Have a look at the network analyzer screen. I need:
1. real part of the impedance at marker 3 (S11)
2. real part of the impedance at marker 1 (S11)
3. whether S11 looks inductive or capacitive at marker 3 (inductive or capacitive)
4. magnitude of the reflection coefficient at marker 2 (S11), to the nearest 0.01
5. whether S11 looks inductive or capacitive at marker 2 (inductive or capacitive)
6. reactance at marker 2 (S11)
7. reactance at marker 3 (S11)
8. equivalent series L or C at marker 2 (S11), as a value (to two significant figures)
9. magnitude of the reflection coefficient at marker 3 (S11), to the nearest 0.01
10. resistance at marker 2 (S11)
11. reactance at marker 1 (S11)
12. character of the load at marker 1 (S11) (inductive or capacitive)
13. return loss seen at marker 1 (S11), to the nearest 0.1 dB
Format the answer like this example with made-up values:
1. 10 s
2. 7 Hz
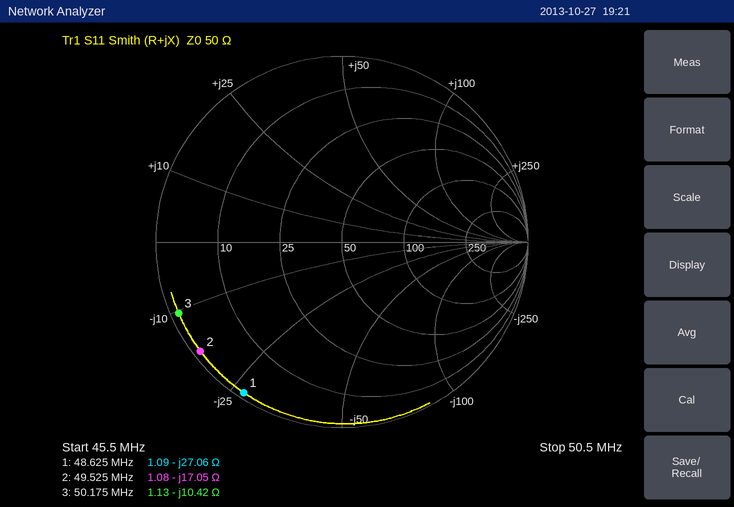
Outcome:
1. 1.13 Ω
2. 1.09 Ω
3. capacitive
4. 0.96
5. capacitive
6. -17.05 Ω
7. -10.42 Ω
8. 190 pF
9. 0.96
10. 1.08 Ω
11. -27.06 Ω
12. capacitive
13. 0.3 dB
